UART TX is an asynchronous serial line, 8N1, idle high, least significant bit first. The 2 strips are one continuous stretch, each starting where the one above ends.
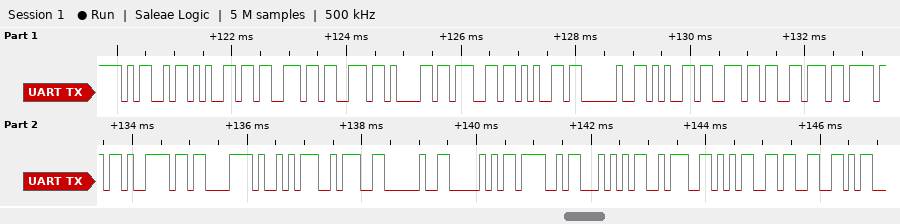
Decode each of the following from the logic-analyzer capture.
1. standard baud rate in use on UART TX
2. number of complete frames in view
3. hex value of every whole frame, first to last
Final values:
9600 baud
23
4D 65 73 73 61 67 65 20 65 6E 76 6F 79 C3 A9 3A 20 50 4F 54 3A 35 33
